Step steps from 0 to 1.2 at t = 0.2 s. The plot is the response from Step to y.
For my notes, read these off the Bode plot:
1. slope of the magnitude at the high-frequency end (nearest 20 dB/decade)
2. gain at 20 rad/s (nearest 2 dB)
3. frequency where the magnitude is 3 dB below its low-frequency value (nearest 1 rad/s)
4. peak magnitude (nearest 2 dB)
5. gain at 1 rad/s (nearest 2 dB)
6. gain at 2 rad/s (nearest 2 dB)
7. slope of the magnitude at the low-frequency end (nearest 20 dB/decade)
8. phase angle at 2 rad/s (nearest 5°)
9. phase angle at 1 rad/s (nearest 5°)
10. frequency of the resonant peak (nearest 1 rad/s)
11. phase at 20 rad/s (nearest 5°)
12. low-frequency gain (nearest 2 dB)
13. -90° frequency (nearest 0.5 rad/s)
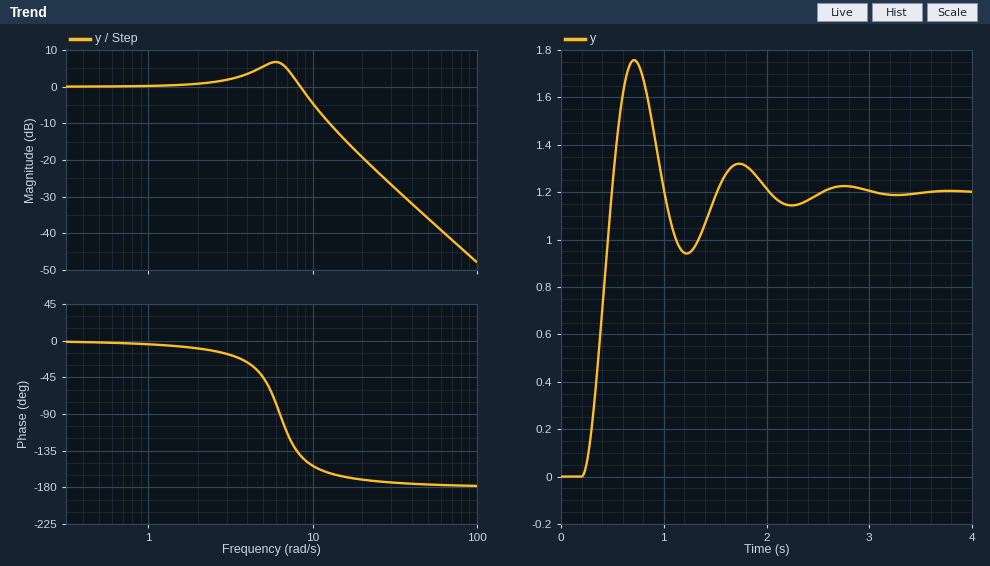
-40 dB/decade
-20 dB
9 rad/s
6 dB
0 dB
0 dB
0 dB/decade
-10°
-5°
6 rad/s
-170°
0 dB
6.5 rad/s
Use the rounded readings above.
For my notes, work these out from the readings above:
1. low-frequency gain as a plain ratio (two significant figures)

1.0
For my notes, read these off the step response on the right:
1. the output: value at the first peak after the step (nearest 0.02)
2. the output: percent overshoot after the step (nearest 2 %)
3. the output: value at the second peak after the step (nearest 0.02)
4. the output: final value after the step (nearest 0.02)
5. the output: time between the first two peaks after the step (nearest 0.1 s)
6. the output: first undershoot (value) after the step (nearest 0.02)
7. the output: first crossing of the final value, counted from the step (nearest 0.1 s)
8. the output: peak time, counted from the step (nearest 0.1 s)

1.76
46 %
1.32
1.20
1.0 s
0.94
0.3 s
0.5 s
